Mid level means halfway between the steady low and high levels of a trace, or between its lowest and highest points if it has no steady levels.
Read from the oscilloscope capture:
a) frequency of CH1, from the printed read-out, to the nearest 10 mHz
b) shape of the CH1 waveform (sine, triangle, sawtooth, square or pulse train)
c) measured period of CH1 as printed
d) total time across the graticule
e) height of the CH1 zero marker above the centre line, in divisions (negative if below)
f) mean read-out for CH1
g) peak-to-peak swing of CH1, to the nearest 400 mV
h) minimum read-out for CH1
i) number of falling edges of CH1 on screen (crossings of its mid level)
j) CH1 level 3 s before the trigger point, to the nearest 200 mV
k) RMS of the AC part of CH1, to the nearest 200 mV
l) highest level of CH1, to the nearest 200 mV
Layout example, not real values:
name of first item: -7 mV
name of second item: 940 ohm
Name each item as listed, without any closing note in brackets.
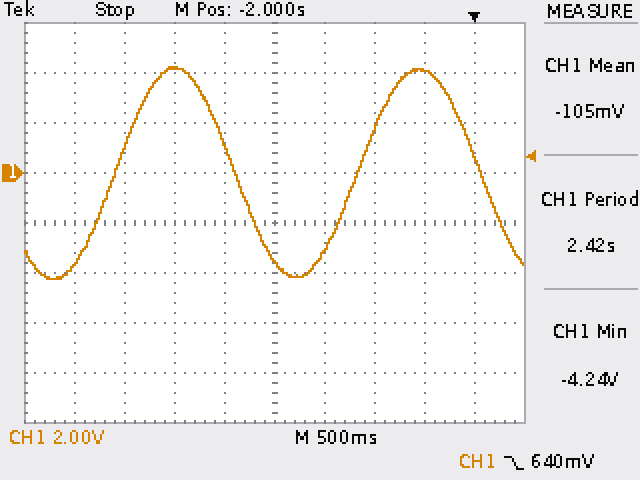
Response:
frequency of CH1, from the printed read-out, to the nearest 10 mHz: 410 mHz
shape of the CH1 waveform: sine
measured period of CH1 as printed: 2.42 s
total time across the graticule: 5 s
height of the CH1 zero marker above the centre line, in divisions: +1.0 div
mean read-out for CH1: -105 mV
peak-to-peak swing of CH1, to the nearest 400 mV: 8.4 V
minimum read-out for CH1: -4.24 V
number of falling edges of CH1 on screen: 2
CH1 level 3 s before the trigger point, to the nearest 200 mV: 4.2 V
RMS of the AC part of CH1, to the nearest 200 mV: 3.0 V
highest level of CH1, to the nearest 200 mV: 4.2 V
